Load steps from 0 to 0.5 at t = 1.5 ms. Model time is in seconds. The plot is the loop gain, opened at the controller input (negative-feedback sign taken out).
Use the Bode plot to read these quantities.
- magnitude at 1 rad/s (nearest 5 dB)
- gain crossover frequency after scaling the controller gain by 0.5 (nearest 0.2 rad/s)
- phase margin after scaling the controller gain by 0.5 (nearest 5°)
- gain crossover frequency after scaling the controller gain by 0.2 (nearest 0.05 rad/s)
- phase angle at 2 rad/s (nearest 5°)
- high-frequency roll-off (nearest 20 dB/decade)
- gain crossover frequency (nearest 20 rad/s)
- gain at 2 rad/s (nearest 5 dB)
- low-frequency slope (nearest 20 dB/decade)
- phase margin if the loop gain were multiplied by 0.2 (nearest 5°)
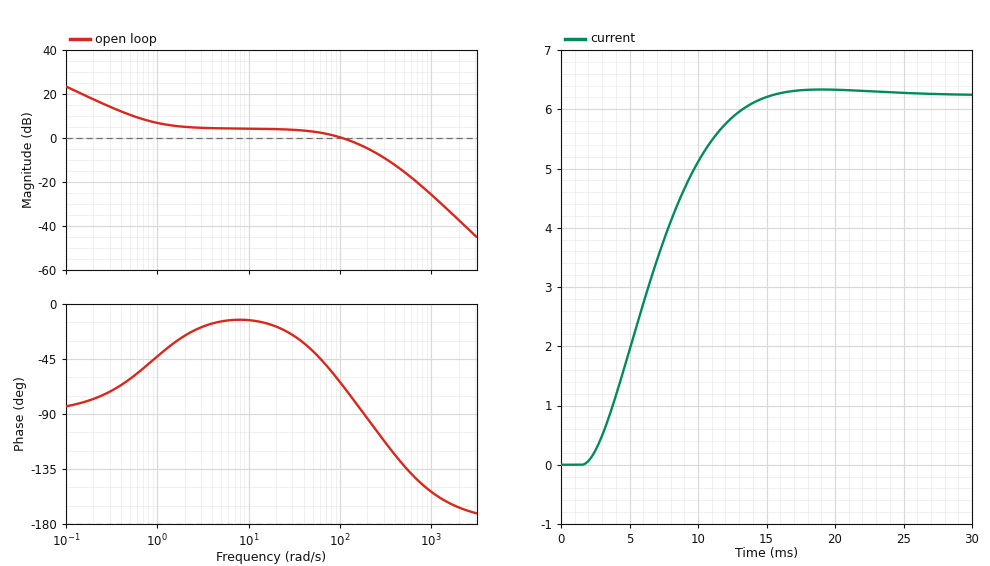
5 dB
1.2 rad/s
145°
0.30 rad/s
-25°
-40 dB/decade
100 rad/s
5 dB
-20 dB/decade
110°
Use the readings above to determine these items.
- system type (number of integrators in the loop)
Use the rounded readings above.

1
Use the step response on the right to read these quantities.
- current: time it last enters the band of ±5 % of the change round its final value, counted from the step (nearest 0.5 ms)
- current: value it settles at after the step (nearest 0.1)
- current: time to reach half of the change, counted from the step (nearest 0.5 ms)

11.5 ms
6.2
5.0 ms
